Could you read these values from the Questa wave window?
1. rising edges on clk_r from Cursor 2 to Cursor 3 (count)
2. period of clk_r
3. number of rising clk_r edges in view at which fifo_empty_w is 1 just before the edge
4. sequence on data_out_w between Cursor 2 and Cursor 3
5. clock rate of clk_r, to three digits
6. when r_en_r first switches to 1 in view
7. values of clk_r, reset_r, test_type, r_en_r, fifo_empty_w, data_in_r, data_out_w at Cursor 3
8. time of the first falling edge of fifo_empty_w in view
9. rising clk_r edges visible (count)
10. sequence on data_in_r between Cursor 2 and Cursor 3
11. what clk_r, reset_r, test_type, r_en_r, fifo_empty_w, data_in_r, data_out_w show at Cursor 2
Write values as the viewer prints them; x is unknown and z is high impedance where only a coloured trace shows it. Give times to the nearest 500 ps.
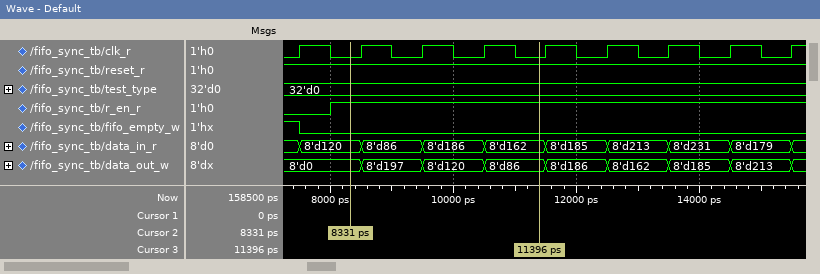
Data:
3
1000 ps
1
8'd0, 8'd197, 8'd120, 8'd86
1.00 GHz
8000 ps
clk_r=0, reset_r=1, test_type=32'd0, r_en_r=1, fifo_empty_w=0, data_in_r=8'd162, data_out_w=8'd86
7500 ps
9
8'd120, 8'd86, 8'd186, 8'd162
clk_r=0, reset_r=1, test_type=32'd0, r_en_r=1, fifo_empty_w=0, data_in_r=8'd120, data_out_w=8'd0
